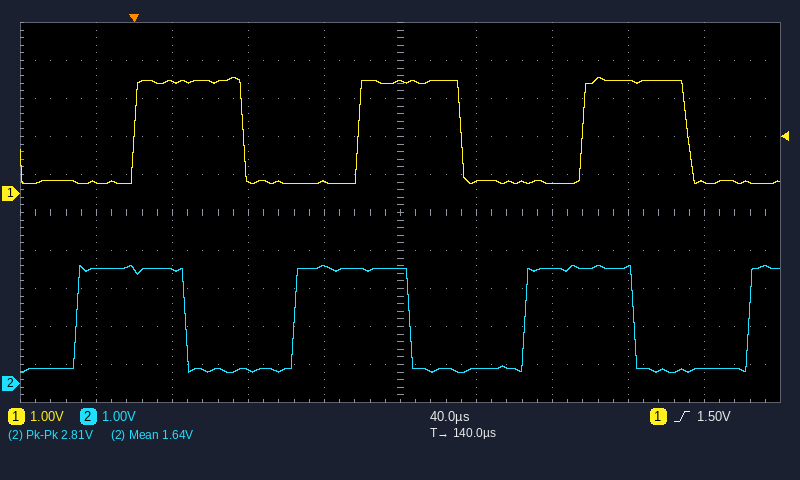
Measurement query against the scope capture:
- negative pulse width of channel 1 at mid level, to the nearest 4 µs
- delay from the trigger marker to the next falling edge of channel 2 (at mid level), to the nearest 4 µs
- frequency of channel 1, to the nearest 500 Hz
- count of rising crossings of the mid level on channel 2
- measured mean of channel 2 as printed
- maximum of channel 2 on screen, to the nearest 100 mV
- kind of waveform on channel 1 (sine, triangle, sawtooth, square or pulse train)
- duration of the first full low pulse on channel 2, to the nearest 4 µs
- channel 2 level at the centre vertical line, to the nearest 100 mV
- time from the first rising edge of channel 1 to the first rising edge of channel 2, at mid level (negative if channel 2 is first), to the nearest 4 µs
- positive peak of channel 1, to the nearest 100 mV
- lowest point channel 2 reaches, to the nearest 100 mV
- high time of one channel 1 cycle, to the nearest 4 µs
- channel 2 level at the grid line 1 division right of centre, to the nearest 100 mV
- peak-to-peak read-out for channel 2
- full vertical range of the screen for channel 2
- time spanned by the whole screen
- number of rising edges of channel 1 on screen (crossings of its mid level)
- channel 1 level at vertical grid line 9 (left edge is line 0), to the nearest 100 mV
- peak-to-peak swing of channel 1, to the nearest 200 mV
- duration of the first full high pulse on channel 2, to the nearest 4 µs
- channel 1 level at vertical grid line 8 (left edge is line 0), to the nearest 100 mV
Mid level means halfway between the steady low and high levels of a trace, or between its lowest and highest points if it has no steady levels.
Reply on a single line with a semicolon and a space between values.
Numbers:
64 µs; 28 µs; 8.5 kHz; 4; 1.64 V; 3.1 V; square; 56 µs; 3.0 V; -32 µs; 3.1 V; 300 mV; 56 µs; 400 mV; 2.81 V; 10 V; 400 µs; 3; 300 mV; 2.8 V; 56 µs; 3.0 V
